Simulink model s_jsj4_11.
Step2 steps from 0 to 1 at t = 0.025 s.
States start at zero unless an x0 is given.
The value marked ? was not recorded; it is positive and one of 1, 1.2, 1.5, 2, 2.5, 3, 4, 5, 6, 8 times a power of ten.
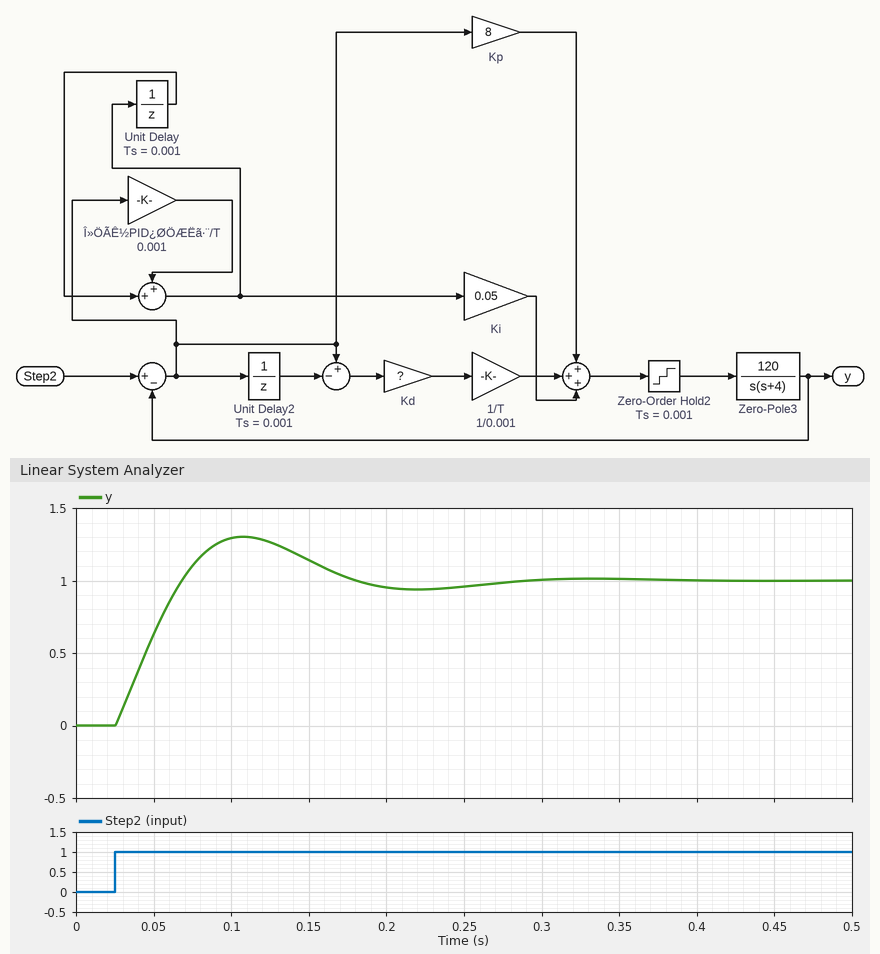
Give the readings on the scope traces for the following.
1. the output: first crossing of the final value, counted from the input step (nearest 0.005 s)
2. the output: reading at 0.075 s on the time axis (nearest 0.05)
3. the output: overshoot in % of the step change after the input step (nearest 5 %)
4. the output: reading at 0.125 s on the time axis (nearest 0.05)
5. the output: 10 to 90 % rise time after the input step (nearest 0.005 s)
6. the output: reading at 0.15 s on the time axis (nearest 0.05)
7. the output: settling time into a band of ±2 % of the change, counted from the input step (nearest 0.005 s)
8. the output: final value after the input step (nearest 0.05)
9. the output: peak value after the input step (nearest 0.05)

0.045 s
1.10
30 %
1.25
0.035 s
1.15
0.245 s
1.00
1.30
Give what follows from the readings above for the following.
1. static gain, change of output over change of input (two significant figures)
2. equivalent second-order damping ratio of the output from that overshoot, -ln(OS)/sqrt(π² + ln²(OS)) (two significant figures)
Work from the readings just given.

1.0
0.36
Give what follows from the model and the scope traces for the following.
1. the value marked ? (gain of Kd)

0.2
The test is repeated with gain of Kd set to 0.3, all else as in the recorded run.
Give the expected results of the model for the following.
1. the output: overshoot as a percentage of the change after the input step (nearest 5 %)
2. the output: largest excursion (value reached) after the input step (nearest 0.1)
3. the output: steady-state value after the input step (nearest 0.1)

20 %
1.2
1.0
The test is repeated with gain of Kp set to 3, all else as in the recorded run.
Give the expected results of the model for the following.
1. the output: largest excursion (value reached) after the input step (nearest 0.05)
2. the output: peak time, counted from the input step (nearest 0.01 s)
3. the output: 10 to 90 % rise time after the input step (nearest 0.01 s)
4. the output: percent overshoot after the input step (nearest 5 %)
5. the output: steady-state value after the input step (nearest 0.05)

1.15
0.13 s
0.05 s
15 %
1.00
